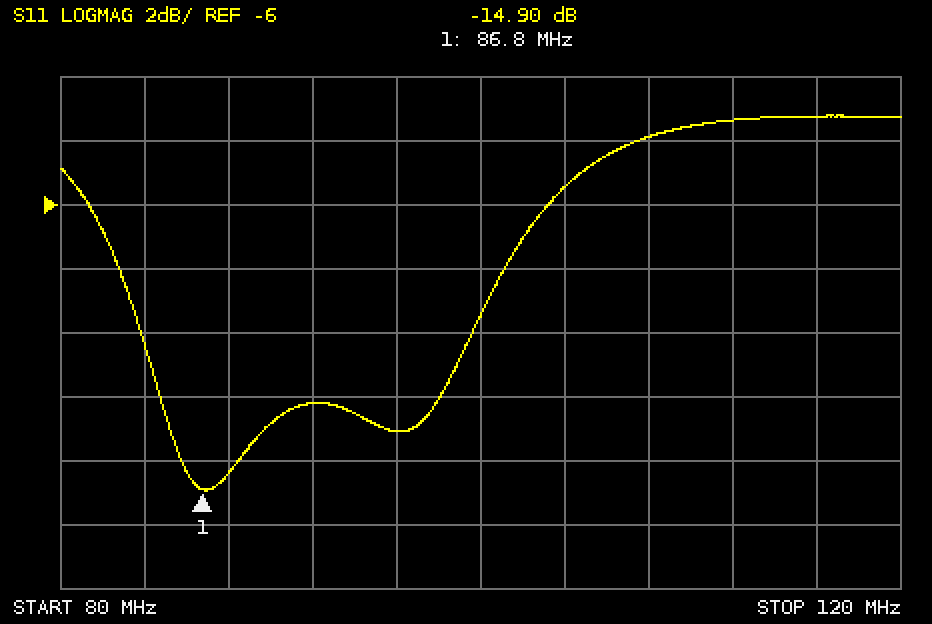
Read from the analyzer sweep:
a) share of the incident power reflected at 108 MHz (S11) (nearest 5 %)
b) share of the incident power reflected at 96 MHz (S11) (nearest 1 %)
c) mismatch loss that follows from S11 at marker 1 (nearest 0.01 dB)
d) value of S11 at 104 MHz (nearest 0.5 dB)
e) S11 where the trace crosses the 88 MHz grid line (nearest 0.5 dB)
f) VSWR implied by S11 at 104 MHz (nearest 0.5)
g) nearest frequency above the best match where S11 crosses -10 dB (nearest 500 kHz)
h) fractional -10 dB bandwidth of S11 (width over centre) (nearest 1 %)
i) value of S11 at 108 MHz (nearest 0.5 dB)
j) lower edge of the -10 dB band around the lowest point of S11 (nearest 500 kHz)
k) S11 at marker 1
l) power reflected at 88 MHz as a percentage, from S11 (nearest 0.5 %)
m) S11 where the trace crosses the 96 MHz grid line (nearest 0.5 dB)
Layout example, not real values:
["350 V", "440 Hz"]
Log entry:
["40 %", "5 %", "0.14 dB", "-5.5 dB", "-14.5 dB", "3.5", "99.5 MHz", "17 %", "-4.0 dB", "84.0 MHz", "-14.90 dB", "3.5 %", "-13.0 dB"]
